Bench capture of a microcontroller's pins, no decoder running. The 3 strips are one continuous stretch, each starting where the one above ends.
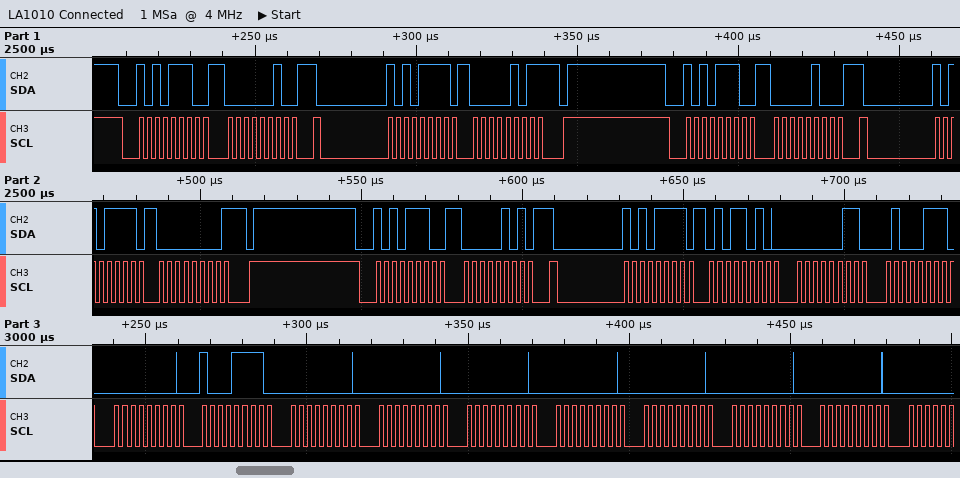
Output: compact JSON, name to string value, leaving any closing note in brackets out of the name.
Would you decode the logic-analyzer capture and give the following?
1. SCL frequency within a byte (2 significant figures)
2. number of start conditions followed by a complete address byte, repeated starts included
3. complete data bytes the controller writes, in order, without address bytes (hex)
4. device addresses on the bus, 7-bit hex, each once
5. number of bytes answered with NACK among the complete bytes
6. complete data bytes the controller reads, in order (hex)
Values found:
{"SCL frequency within a byte": "400 kHz", "number of start conditions followed by a complete address byte, repeated starts included": "6", "complete data bytes the controller writes, in order, without address bytes": "02 04 05", "device addresses on the bus, 7-bit hex, each once": "0x57", "number of bytes answered with NACK among the complete bytes": "2", "complete data bytes the controller reads, in order": "05 00 5A 03 47 00 8F 00 00 00 00 00 00 00"}
